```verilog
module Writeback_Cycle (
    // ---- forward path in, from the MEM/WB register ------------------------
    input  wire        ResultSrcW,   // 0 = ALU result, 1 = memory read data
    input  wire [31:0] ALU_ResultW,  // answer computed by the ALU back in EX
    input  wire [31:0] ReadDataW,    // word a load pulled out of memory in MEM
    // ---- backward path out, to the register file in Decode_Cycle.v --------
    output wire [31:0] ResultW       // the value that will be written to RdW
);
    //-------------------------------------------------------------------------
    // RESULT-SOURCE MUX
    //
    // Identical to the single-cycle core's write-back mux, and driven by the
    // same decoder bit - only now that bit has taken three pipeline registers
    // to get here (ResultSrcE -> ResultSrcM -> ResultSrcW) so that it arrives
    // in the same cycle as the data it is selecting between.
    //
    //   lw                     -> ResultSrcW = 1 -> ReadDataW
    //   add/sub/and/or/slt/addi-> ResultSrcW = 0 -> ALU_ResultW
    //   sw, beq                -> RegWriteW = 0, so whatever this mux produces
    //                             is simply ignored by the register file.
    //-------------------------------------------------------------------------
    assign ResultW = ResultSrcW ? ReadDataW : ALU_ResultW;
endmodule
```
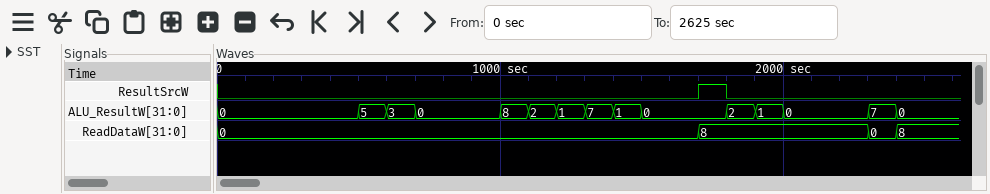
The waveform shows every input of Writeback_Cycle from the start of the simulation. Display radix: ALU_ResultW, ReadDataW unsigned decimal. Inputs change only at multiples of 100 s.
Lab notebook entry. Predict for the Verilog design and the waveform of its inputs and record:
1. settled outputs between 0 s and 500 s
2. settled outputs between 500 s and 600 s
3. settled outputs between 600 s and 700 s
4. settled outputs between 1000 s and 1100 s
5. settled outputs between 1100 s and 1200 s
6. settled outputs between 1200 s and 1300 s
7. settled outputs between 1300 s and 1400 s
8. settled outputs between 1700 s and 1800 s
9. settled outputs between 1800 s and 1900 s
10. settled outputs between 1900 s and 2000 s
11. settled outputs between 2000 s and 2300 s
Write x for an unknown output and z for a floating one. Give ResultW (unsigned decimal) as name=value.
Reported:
ResultW=0
ResultW=5
ResultW=3
ResultW=8
ResultW=2
ResultW=1
ResultW=7
ResultW=8
ResultW=2
ResultW=1
ResultW=0
